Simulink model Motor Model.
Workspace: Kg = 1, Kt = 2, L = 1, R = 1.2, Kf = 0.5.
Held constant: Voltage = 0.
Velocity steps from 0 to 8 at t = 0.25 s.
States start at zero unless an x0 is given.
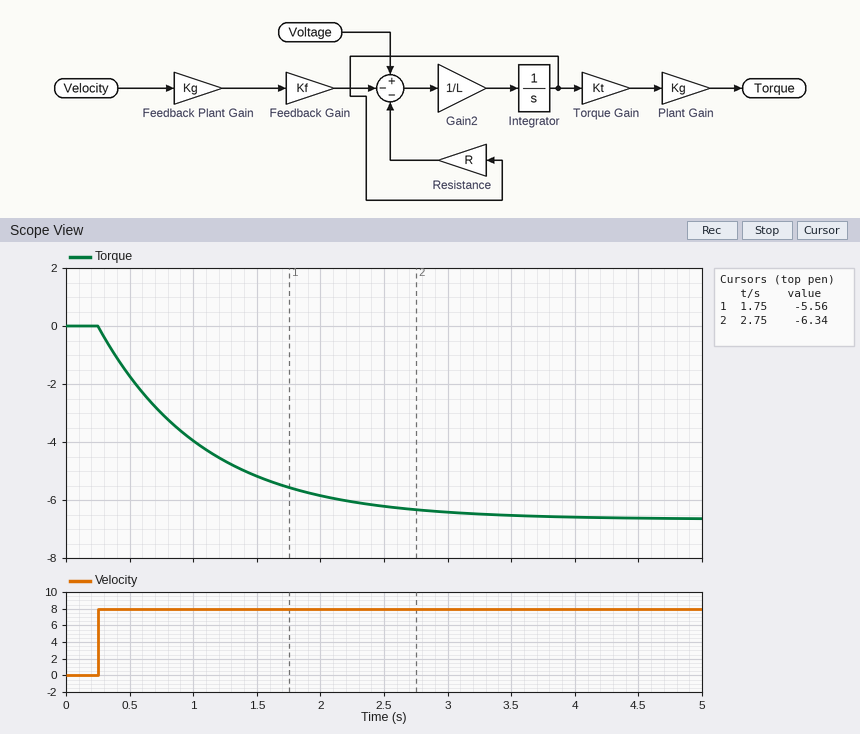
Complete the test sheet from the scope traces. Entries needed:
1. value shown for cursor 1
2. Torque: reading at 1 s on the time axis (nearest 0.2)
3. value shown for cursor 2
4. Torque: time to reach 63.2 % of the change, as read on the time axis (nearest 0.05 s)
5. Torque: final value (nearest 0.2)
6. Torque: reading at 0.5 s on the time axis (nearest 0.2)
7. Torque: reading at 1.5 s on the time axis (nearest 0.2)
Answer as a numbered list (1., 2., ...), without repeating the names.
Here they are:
1. -5.56
2. -4.0
3. -6.34
4. 1.10 s
5. -6.6
6. -1.8
7. -5.2
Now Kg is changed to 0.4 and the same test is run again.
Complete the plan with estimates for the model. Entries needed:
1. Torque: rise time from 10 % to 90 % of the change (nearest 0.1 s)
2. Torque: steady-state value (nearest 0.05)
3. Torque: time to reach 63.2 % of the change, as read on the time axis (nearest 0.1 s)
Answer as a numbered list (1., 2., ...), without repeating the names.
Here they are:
1. 1.8 s
2. -1.05
3. 1.1 s
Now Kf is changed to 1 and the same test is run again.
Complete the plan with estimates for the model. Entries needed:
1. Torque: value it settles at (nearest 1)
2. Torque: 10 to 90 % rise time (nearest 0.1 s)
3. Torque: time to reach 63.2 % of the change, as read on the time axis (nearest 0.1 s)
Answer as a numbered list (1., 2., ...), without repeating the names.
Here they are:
1. -13
2. 1.8 s
3. 1.1 s
